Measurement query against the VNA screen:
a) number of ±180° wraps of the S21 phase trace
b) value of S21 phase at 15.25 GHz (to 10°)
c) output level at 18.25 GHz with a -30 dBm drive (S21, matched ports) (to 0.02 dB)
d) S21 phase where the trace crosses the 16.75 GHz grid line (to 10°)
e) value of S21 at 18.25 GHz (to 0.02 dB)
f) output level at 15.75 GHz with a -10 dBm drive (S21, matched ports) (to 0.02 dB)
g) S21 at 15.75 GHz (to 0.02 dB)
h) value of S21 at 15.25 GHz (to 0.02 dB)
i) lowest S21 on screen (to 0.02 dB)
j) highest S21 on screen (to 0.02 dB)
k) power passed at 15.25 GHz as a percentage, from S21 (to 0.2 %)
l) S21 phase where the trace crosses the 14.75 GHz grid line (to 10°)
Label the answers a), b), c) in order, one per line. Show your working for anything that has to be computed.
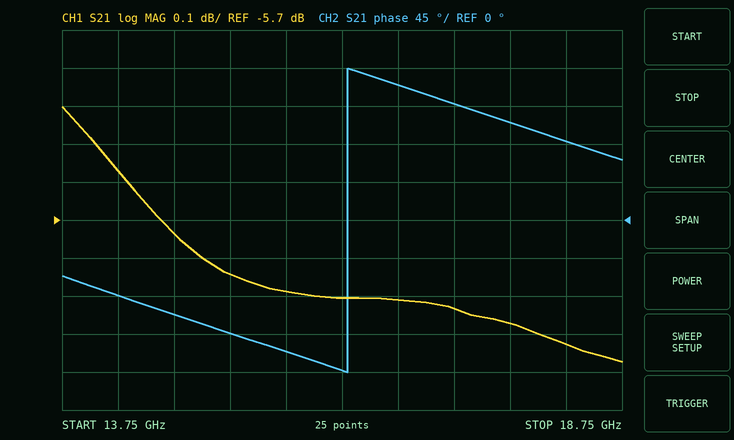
a) 1
b) -130°
c) -30 dBm + (-6.02 dB) = -36.02 dBm
d) 160°
e) -6.02 dB
f) -10 dBm + (-5.88 dB) = -15.88 dBm
g) -5.88 dB
h) -5.84 dB
i) -6.08 dB
j) -5.40 dB
k) 10^(-5.84/10) ≈ 26.1 %, so 26.0 % to the nearest 0.2 %
l) -110°
